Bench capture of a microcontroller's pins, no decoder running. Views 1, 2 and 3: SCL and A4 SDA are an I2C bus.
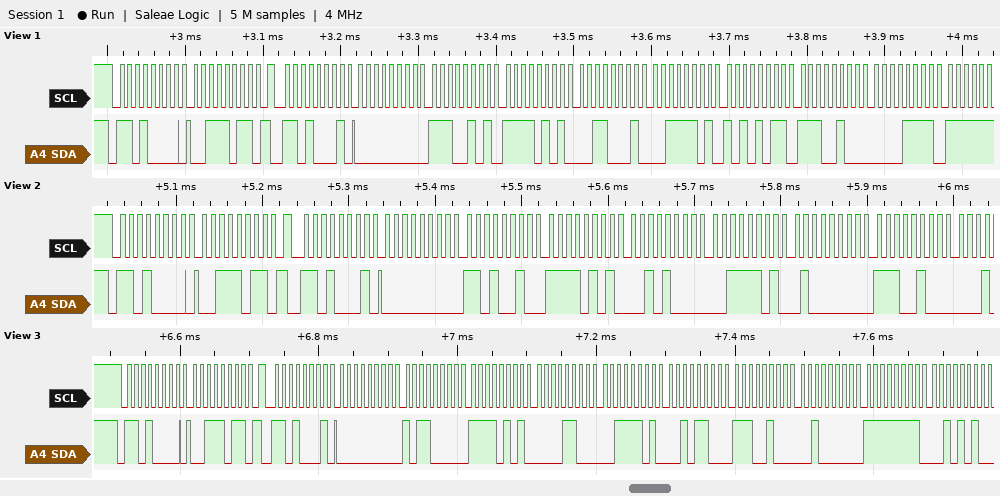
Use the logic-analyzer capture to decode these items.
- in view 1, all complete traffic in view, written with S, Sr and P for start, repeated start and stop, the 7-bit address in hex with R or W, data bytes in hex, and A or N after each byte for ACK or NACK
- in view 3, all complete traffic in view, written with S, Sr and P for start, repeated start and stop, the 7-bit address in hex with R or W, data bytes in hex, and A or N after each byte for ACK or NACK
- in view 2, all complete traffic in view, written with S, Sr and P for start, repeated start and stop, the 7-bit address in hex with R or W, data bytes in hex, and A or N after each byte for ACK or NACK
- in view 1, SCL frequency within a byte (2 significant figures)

S 68W A 3B A Sr 68R A 00 A E5 A F5 A 31 A 3D A AB A E4 A 0F A
S 68W A 3B A Sr 68R A 00 A B0 A F5 A 0C A 3D A 2C A E4 A 20 A FF A 2A A
S 68W A 3B A Sr 68R A 00 A D2 A F5 A 28 A 3D A 40 A E4 A
100 kHz
